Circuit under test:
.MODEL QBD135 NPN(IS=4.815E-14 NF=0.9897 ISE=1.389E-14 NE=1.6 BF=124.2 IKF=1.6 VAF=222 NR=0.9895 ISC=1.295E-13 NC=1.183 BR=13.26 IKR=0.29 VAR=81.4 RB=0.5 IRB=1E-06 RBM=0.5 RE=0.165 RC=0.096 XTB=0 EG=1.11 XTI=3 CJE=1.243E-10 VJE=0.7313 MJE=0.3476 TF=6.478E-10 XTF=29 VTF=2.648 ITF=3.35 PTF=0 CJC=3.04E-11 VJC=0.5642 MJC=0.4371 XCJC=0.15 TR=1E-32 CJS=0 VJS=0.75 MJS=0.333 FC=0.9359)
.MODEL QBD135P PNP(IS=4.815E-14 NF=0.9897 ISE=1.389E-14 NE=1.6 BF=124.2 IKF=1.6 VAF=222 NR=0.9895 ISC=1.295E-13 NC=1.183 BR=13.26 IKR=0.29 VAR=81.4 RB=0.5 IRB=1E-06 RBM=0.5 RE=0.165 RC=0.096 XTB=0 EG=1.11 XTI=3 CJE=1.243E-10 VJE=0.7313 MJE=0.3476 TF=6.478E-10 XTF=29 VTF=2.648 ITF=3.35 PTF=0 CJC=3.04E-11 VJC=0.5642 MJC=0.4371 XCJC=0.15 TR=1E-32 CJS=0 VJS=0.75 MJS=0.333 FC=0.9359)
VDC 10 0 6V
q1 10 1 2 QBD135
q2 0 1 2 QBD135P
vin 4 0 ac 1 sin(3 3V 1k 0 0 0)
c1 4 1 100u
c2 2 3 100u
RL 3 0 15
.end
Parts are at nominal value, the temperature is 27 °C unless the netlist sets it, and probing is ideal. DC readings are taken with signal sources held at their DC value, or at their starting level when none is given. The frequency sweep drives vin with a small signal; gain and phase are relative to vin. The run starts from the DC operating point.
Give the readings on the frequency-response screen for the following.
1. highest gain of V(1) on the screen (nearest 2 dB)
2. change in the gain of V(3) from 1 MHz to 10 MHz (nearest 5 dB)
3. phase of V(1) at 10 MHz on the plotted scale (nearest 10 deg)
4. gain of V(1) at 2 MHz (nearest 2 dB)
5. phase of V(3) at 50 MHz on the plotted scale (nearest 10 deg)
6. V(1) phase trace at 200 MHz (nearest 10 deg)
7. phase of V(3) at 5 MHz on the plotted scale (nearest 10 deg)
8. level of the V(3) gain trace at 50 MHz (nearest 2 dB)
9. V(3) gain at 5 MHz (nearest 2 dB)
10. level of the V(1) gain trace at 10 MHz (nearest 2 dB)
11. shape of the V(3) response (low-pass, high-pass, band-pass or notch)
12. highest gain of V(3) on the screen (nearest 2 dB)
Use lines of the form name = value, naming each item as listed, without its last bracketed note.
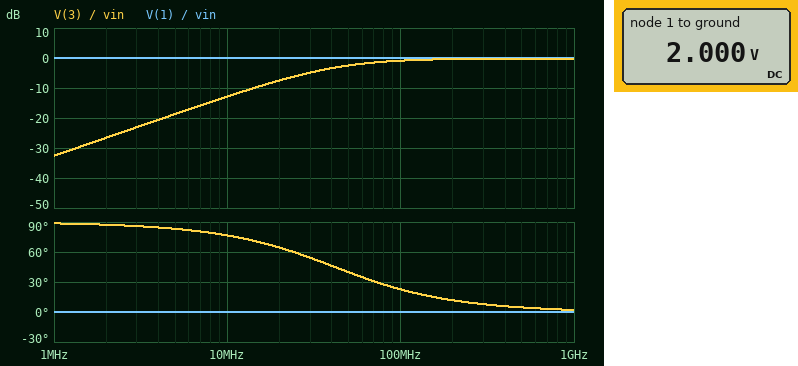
highest gain of V(1) on the screen = 0 dB
change in the gain of V(3) from 1 MHz to 10 MHz = 20 dB
phase of V(1) at 10 MHz on the plotted scale = 0 deg
gain of V(1) at 2 MHz = 0 dB
phase of V(3) at 50 MHz on the plotted scale = 40 deg
V(1) phase trace at 200 MHz = 0 deg
phase of V(3) at 5 MHz on the plotted scale = 80 deg
level of the V(3) gain trace at 50 MHz = -2 dB
V(3) gain at 5 MHz = -18 dB
level of the V(1) gain trace at 10 MHz = 0 dB
shape of the V(3) response = high-pass
highest gain of V(3) on the screen = 0 dB
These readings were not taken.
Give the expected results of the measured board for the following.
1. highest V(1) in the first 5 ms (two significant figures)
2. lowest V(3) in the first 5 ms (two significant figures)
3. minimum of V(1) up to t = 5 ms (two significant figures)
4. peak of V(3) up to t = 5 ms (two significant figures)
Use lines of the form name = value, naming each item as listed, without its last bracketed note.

highest V(1) in the first 5 ms = 5.2 V
lowest V(3) in the first 5 ms = -2.2 V
minimum of V(1) up to t = 5 ms = -910 mV
peak of V(3) up to t = 5 ms = 2.3 V
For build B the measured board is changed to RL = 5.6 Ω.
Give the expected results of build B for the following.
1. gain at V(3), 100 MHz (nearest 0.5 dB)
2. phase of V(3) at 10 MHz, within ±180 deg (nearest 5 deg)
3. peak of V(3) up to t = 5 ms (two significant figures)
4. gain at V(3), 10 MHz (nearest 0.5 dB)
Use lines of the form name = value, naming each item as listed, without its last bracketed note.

gain at V(3), 100 MHz = -4.0 dB
phase of V(3) at 10 MHz, within ±180 deg = 85 deg
peak of V(3) up to t = 5 ms = 2.1 V
gain at V(3), 10 MHz = -21.0 dB
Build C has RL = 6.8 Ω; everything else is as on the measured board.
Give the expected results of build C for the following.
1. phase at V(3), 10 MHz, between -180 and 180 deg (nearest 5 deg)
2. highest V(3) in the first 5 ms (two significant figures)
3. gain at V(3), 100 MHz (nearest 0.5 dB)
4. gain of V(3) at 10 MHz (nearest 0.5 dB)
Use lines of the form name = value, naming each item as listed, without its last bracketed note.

phase at V(3), 10 MHz, between -180 and 180 deg = 85 deg
highest V(3) in the first 5 ms = 2.2 V
gain at V(3), 100 MHz = -3.0 dB
gain of V(3) at 10 MHz = -19.5 dB
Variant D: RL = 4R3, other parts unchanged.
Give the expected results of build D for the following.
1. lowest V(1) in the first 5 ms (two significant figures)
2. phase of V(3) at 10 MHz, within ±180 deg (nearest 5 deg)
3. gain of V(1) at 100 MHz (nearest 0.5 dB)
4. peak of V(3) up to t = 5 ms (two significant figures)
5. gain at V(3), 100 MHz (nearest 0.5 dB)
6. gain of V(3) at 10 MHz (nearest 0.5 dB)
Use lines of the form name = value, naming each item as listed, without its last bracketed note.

lowest V(1) in the first 5 ms = -900 mV
phase of V(3) at 10 MHz, within ±180 deg = 85 deg
gain of V(1) at 100 MHz = 0 dB
peak of V(3) up to t = 5 ms = 2.1 V
gain at V(3), 100 MHz = -5.5 dB
gain of V(3) at 10 MHz = -23.5 dB
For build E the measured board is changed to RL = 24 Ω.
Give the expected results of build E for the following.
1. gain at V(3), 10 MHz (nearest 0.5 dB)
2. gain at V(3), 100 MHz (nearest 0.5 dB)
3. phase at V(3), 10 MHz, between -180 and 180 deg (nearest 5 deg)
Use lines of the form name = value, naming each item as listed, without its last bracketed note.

gain at V(3), 10 MHz = -9.0 dB
gain at V(3), 100 MHz = -0.5 dB
phase at V(3), 10 MHz, between -180 and 180 deg = 70 deg
